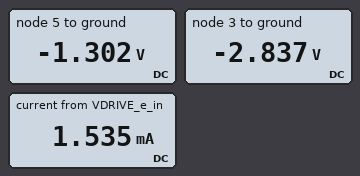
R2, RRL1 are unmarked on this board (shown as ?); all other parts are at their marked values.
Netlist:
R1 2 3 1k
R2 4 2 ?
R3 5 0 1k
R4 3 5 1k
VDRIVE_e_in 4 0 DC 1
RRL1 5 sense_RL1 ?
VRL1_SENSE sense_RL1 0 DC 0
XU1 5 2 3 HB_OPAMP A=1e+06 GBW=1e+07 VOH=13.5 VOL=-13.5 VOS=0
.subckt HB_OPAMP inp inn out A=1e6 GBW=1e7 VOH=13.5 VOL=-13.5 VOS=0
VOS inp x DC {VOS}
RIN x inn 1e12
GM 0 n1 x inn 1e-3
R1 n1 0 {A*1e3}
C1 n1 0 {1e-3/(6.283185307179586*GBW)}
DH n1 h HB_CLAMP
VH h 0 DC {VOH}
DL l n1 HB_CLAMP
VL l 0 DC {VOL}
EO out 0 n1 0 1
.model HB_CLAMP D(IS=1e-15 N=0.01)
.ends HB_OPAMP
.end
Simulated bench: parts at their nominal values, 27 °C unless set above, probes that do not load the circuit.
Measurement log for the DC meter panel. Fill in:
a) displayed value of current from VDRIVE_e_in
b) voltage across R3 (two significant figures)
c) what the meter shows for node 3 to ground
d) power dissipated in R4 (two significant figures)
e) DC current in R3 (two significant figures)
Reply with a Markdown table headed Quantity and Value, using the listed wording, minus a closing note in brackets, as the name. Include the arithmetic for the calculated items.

| Quantity | Value |
|---|---|
| displayed value of current from VDRIVE_e_in | 1.535 mA |
| voltage across R3 | 0 V - (-1.302 V) = 1.3 V |
| what the meter shows for node 3 to ground | -2.837 V |
| power dissipated in R4 | (-1.302 V - (-2.837 V))^2 / 1 kΩ = 2.4 mW |
| DC current in R3 | (0 V - (-1.302 V)) / 1 kΩ = 1.3 mA |
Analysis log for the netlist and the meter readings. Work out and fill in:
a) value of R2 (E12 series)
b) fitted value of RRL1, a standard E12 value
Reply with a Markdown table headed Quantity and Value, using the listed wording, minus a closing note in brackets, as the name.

| Quantity | Value |
|---|---|
| value of R2 | 1.5 kΩ |
| fitted value of RRL1, a standard E12 value | 5.6 kΩ |
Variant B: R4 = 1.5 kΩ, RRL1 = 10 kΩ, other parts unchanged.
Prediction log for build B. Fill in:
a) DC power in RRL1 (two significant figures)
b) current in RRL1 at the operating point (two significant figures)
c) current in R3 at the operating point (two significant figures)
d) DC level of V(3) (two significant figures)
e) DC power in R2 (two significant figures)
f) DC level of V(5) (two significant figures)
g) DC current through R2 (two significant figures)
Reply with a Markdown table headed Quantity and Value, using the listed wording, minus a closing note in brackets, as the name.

| Quantity | Value |
|---|---|
| DC power in RRL1 | 46 µW |
| current in RRL1 at the operating point | 68 µA |
| current in R3 at the operating point | 680 µA |
| DC level of V(3) | -1.8 V |
| DC power in R2 | 1.9 mW |
| DC level of V(5) | -680 mV |
| DC current through R2 | 1.1 mA |
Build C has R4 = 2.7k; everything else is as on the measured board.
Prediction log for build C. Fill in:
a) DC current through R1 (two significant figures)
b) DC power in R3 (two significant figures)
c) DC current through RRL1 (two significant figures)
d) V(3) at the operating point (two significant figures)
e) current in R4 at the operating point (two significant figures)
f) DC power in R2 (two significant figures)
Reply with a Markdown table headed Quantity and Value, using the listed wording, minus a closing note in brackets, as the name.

| Quantity | Value |
|---|---|
| DC current through R1 | 840 µA |
| DC power in R3 | 70 µW |
| DC current through RRL1 | 47 µA |
| V(3) at the operating point | -1.1 V |
| current in R4 at the operating point | 310 µA |
| DC power in R2 | 1.1 mW |
